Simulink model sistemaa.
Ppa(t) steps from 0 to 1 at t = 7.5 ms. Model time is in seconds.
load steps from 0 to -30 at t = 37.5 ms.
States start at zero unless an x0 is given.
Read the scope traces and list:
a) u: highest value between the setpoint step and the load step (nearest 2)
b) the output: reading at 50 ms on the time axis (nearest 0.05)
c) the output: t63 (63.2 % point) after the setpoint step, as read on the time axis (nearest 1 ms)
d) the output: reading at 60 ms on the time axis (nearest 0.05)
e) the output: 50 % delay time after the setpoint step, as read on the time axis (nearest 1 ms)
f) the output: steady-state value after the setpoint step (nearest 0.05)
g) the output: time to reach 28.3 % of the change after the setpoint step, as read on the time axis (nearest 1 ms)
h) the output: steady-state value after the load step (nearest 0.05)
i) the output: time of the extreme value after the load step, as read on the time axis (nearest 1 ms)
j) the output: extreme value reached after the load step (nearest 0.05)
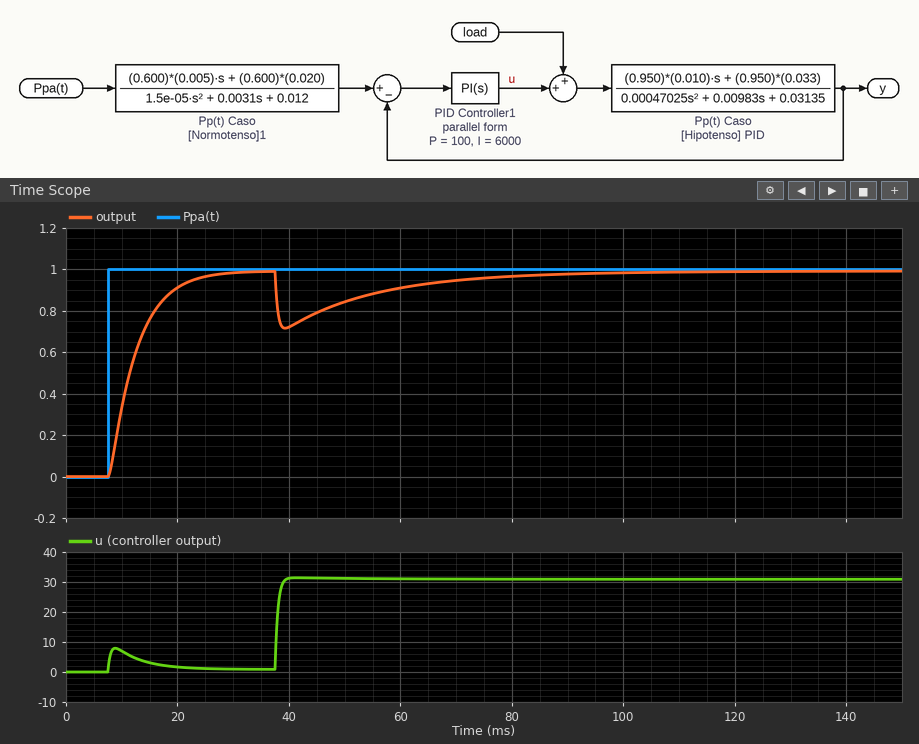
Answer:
8
0.85
13 ms
0.90
11 ms
1.00
10 ms
1.00
39 ms
0.70
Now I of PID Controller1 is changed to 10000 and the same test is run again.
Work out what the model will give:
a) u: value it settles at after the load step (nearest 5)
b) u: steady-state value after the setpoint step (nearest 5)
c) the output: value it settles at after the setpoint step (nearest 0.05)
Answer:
30
0
1.00
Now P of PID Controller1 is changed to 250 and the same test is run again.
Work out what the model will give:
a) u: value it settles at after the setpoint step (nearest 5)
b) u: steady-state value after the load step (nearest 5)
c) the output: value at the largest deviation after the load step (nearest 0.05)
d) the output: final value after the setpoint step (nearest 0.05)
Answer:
0
30
0.85
1.00
